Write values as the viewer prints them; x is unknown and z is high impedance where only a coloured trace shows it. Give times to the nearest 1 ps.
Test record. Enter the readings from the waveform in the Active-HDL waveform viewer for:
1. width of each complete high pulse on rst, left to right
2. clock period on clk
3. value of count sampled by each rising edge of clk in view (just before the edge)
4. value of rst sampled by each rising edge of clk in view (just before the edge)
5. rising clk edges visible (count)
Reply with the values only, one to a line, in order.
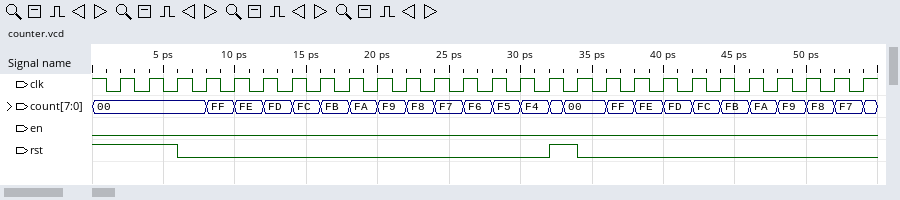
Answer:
2 ps
2 ps
00, 00, 00, 00, FF, FE, FD, FC, FB, FA, F9, F8, F7, F6, F5, F4, 00, 00, FF, FE, FD, FC, FB, FA, F9, F8, F7
1 1 1 0 0 0 0 0 0 0 0 0 0 0 0 0 1 0 0 0 0 0 0 0 0 0 0
27
